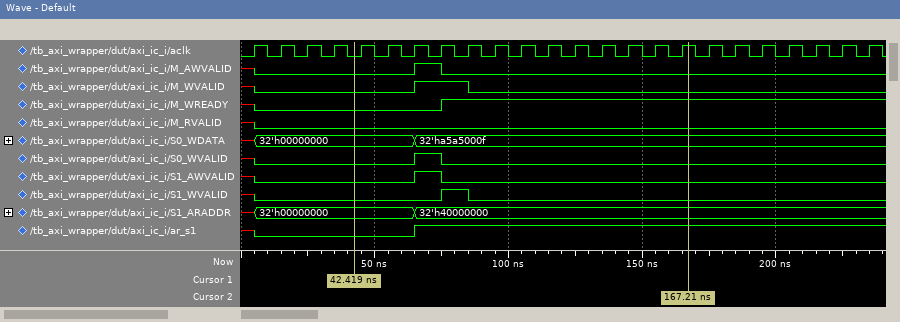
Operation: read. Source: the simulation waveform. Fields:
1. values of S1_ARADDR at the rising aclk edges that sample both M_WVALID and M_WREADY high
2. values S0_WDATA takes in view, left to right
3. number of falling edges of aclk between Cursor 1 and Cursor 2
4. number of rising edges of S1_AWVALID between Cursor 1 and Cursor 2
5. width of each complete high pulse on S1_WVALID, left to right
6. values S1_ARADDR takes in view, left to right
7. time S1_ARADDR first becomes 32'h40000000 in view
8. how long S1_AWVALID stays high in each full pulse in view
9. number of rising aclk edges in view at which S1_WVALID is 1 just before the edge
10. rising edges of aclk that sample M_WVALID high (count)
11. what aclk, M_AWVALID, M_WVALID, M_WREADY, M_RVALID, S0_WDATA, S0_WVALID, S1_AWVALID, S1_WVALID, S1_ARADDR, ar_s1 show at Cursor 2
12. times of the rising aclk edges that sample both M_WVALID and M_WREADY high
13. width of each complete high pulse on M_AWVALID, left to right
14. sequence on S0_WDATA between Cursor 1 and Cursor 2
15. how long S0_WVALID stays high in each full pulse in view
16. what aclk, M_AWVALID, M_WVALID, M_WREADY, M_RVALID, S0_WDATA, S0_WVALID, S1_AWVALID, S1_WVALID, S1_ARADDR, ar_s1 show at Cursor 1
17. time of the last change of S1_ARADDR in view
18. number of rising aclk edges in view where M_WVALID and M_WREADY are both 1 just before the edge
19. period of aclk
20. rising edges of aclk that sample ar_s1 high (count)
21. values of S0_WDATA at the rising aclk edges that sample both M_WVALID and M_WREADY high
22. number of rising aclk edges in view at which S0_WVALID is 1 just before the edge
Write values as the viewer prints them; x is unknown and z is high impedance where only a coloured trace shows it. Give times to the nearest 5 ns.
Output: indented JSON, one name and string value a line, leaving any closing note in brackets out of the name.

{
  "values of S1_ARADDR at the rising aclk edges that sample both M_WVALID and M_WREADY high": "32'h40000000",
  "values S0_WDATA takes in view, left to right": "x, 32'h00000000, 32'ha5a5000f",
  "number of falling edges of aclk between Cursor 1 and Cursor 2": "12",
  "number of rising edges of S1_AWVALID between Cursor 1 and Cursor 2": "1",
  "width of each complete high pulse on S1_WVALID, left to right": "10 ns",
  "values S1_ARADDR takes in view, left to right": "x, 32'h00000000, 32'h40000000",
  "time S1_ARADDR first becomes 32'h40000000 in view": "65 ns",
  "how long S1_AWVALID stays high in each full pulse in view": "10 ns",
  "number of rising aclk edges in view at which S1_WVALID is 1 just before the edge": "1",
  "rising edges of aclk that sample M_WVALID high": "2",
  "what aclk, M_AWVALID, M_WVALID, M_WREADY, M_RVALID, S0_WDATA, S0_WVALID, S1_AWVALID, S1_WVALID, S1_ARADDR, ar_s1 show at Cursor 2": "aclk=1, M_AWVALID=0, M_WVALID=0, M_WREADY=1, M_RVALID=0, S0_WDATA=32'ha5a5000f, S0_WVALID=0, S1_AWVALID=0, S1_WVALID=0, S1_ARADDR=32'h40000000, ar_s1=1",
  "times of the rising aclk edges that sample both M_WVALID and M_WREADY high": "85 ns",
  "width of each complete high pulse on M_AWVALID, left to right": "10 ns",
  "sequence on S0_WDATA between Cursor 1 and Cursor 2": "32'h00000000, 32'ha5a5000f",
  "how long S0_WVALID stays high in each full pulse in view": "10 ns",
  "what aclk, M_AWVALID, M_WVALID, M_WREADY, M_RVALID, S0_WDATA, S0_WVALID, S1_AWVALID, S1_WVALID, S1_ARADDR, ar_s1 show at Cursor 1": "aclk=0, M_AWVALID=0, M_WVALID=0, M_WREADY=0, M_RVALID=0, S0_WDATA=32'h00000000, S0_WVALID=0, S1_AWVALID=0, S1_WVALID=0, S1_ARADDR=32'h00000000, ar_s1=0",
  "time of the last change of S1_ARADDR in view": "65 ns",
  "number of rising aclk edges in view where M_WVALID and M_WREADY are both 1 just before the edge": "1",
  "period of aclk": "10 ns",
  "rising edges of aclk that sample ar_s1 high": "17",
  "values of S0_WDATA at the rising aclk edges that sample both M_WVALID and M_WREADY high": "32'ha5a5000f",
  "number of rising aclk edges in view at which S0_WVALID is 1 just before the edge": "1"
}
